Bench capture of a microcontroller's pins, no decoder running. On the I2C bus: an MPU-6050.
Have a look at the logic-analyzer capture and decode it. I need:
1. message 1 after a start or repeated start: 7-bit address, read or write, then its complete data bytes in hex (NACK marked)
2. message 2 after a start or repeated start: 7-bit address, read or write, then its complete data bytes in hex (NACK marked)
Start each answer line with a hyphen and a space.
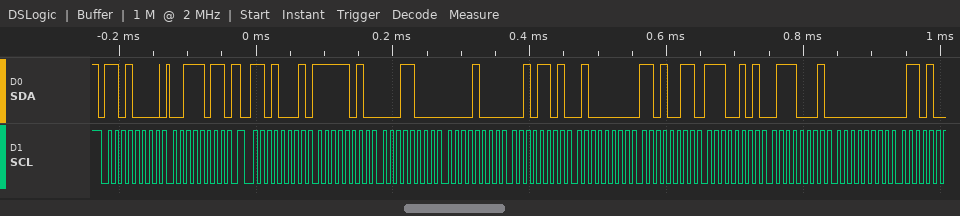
- 0x68 write: 3B
- 0x68 read: FA 18 08 2D 40 D3 E5 71 00
